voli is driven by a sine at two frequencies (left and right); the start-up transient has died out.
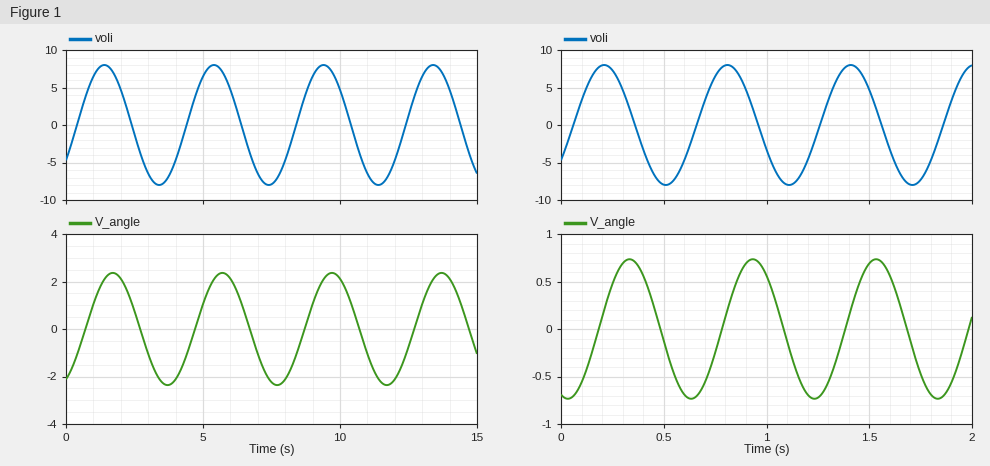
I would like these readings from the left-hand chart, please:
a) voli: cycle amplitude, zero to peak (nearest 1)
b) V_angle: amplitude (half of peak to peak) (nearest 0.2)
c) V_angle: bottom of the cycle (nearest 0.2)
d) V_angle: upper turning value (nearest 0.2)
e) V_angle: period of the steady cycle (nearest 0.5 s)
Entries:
8
2.4
-2.4
2.4
4.0 s
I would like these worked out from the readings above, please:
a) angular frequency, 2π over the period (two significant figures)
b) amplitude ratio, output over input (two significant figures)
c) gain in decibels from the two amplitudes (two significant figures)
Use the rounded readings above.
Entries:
1.6 rad/s
0.30
-10 dB
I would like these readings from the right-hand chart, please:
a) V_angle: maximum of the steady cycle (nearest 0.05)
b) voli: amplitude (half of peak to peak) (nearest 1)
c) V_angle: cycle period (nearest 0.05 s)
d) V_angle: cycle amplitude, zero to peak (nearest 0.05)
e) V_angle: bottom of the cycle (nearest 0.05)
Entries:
0.75
8
0.60 s
0.75
-0.75
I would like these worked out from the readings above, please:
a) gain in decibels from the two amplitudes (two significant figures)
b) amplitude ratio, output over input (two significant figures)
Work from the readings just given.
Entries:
-21 dB
0.094
